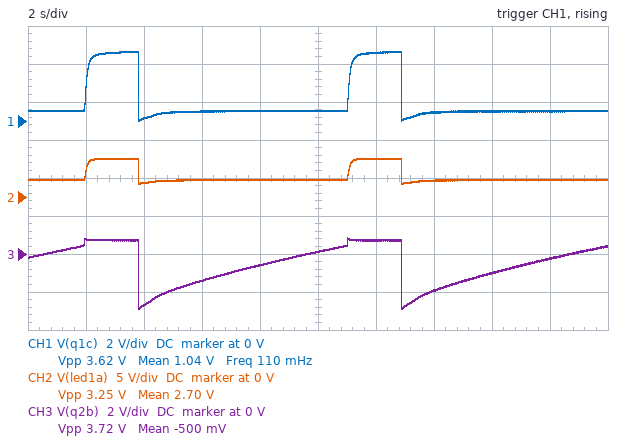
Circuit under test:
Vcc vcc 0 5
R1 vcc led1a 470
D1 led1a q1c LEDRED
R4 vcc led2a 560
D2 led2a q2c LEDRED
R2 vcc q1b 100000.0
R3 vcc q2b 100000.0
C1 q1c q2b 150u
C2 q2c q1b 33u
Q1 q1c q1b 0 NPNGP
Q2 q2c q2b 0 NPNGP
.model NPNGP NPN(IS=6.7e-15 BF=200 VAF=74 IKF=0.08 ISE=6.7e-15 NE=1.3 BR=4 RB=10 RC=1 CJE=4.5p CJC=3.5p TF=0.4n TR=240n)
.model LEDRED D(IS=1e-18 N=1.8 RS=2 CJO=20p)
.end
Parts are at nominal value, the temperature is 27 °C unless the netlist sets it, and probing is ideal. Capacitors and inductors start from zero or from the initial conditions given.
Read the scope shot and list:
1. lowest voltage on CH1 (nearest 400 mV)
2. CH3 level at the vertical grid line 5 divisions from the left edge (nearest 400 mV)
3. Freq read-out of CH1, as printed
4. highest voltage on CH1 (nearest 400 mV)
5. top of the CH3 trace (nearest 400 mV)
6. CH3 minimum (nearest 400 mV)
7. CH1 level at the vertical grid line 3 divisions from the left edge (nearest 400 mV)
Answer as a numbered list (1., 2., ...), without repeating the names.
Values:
1. 0 V
2. 0 V
3. 110 mHz
4. 3.6 V
5. 800 mV
6. -2.8 V
7. 400 mV
